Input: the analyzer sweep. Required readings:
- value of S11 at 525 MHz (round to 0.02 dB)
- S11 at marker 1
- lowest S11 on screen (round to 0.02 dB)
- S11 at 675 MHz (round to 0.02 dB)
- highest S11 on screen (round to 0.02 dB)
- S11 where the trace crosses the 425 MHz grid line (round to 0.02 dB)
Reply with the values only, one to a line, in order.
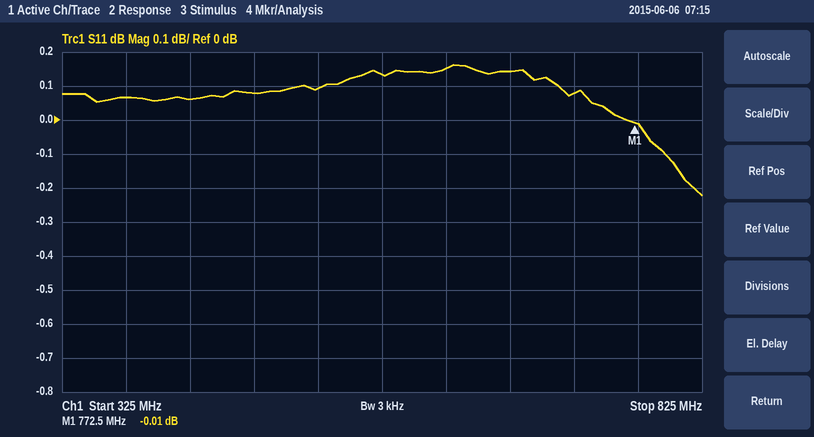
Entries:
0.10 dB
-0.01 dB
-0.22 dB
0.14 dB
0.16 dB
0.06 dB
